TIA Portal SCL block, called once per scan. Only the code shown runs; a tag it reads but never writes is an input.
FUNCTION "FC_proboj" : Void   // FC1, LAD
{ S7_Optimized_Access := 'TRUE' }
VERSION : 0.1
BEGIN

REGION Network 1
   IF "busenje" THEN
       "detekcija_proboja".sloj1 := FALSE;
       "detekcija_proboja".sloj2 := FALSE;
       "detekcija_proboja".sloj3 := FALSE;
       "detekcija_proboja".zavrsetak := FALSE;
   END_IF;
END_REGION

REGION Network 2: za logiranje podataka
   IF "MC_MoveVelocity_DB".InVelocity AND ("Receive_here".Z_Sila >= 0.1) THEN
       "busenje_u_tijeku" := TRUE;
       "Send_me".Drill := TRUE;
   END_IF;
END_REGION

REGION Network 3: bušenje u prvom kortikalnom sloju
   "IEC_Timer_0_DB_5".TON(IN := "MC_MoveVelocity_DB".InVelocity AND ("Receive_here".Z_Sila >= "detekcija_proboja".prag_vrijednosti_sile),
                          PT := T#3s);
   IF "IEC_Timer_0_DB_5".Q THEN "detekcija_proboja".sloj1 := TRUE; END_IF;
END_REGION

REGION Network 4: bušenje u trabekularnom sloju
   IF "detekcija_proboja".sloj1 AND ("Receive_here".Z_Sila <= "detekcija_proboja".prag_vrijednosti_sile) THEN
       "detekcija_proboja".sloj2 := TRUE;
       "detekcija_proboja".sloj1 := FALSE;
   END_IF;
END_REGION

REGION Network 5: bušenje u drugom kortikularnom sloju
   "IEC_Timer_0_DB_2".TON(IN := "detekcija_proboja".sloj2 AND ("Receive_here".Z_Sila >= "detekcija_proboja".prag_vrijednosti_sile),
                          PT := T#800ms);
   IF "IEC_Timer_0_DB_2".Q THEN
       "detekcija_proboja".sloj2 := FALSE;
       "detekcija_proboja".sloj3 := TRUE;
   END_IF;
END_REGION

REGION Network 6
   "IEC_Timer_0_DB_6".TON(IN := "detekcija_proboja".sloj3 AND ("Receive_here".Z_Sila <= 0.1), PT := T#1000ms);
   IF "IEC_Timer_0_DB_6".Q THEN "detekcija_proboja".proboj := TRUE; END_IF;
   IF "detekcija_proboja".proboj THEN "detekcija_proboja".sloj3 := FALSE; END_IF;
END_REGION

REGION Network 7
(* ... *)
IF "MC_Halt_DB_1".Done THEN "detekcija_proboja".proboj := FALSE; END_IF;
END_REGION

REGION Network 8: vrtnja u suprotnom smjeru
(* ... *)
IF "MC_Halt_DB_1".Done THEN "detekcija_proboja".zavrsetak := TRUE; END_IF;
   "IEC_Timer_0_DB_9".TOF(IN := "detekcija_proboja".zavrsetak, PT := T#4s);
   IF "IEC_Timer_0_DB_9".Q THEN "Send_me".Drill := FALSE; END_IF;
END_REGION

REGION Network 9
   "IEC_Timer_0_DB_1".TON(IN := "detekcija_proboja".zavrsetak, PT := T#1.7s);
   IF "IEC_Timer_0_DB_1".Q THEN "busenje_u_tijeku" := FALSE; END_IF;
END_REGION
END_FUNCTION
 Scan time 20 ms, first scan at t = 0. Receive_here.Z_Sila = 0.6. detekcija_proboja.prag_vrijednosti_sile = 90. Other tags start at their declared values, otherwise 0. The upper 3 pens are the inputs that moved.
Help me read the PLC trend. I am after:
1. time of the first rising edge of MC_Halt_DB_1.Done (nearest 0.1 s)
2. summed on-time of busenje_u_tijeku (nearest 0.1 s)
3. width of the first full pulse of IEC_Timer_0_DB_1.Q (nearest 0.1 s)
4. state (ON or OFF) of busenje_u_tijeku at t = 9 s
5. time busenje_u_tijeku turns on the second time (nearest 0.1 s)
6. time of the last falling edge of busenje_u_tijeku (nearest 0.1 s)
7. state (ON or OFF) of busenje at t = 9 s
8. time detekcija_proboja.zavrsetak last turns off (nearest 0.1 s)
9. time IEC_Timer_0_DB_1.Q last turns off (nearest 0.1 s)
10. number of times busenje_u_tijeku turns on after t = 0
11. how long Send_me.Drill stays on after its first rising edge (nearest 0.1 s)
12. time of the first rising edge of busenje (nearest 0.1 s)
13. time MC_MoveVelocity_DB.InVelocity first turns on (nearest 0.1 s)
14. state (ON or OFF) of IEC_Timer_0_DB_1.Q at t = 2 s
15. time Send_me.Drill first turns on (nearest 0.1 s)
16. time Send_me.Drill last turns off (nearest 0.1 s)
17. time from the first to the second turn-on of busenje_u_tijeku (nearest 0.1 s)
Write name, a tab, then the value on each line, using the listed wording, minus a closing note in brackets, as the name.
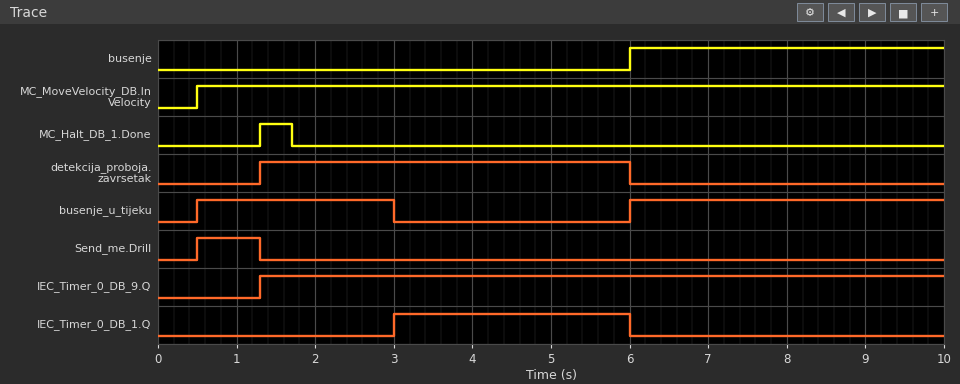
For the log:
time of the first rising edge of MC_Halt_DB_1.Done	1.3 s
summed on-time of busenje_u_tijeku	6.5 s
width of the first full pulse of IEC_Timer_0_DB_1.Q	3.0 s
state (ON or OFF) of busenje_u_tijeku at t = 9 s	ON
time busenje_u_tijeku turns on the second time	6.0 s
time of the last falling edge of busenje_u_tijeku	3.0 s
state (ON or OFF) of busenje at t = 9 s	ON
time detekcija_proboja.zavrsetak last turns off	6.0 s
time IEC_Timer_0_DB_1.Q last turns off	6.0 s
number of times busenje_u_tijeku turns on after t = 0	2
how long Send_me.Drill stays on after its first rising edge	0.8 s
time of the first rising edge of busenje	6.0 s
time MC_MoveVelocity_DB.InVelocity first turns on	0.5 s
state (ON or OFF) of IEC_Timer_0_DB_1.Q at t = 2 s	OFF
time Send_me.Drill first turns on	0.5 s
time Send_me.Drill last turns off	1.3 s
time from the first to the second turn-on of busenje_u_tijeku	5.5 s
